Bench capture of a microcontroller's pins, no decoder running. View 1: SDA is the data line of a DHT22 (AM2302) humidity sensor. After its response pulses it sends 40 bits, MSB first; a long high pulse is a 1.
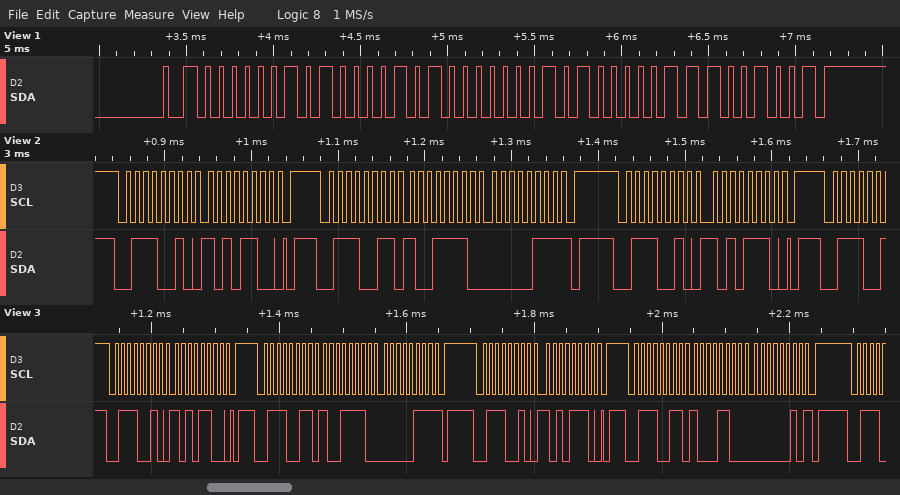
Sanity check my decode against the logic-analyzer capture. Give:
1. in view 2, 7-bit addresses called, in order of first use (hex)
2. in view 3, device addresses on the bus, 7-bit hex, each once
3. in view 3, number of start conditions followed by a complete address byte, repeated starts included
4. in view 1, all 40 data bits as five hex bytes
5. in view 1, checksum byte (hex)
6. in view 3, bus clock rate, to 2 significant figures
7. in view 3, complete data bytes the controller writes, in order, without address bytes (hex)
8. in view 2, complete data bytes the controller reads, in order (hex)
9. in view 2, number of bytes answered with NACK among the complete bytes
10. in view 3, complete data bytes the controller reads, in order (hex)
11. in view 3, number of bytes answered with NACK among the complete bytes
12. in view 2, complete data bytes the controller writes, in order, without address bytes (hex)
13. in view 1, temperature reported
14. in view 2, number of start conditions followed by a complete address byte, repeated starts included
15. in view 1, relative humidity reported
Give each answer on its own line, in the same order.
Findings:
0x39
0x39
4
02 85 01 41 C9
0xC9
100 kHz
AC AE
9E 07
1
9E 07 8C 02
2
AC AE
32.1 °C
3
64.5 %
